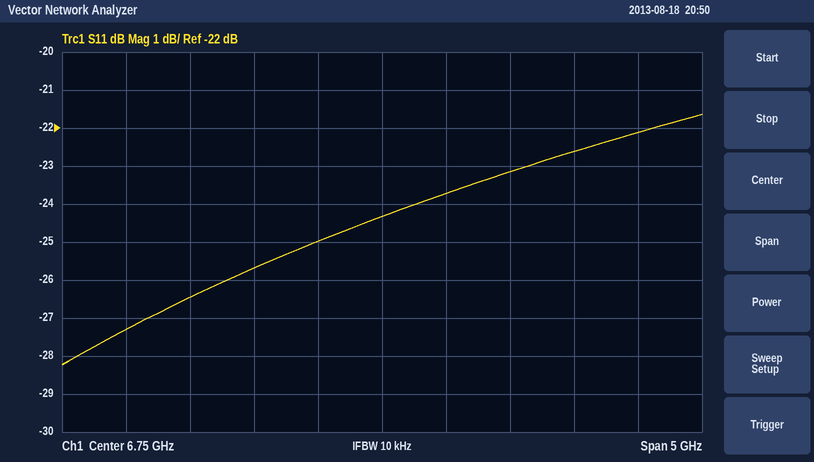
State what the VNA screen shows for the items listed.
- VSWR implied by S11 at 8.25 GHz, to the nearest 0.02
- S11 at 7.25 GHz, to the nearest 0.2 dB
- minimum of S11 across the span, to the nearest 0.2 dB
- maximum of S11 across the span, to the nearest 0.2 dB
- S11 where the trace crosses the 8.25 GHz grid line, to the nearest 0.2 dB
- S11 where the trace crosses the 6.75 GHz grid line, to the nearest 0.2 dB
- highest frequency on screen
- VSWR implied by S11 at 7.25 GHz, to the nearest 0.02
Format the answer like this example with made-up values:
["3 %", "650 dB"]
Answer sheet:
["1.16", "-23.8 dB", "-28.2 dB", "-21.6 dB", "-22.6 dB", "-24.4 dB", "9.25 GHz", "1.14"]
